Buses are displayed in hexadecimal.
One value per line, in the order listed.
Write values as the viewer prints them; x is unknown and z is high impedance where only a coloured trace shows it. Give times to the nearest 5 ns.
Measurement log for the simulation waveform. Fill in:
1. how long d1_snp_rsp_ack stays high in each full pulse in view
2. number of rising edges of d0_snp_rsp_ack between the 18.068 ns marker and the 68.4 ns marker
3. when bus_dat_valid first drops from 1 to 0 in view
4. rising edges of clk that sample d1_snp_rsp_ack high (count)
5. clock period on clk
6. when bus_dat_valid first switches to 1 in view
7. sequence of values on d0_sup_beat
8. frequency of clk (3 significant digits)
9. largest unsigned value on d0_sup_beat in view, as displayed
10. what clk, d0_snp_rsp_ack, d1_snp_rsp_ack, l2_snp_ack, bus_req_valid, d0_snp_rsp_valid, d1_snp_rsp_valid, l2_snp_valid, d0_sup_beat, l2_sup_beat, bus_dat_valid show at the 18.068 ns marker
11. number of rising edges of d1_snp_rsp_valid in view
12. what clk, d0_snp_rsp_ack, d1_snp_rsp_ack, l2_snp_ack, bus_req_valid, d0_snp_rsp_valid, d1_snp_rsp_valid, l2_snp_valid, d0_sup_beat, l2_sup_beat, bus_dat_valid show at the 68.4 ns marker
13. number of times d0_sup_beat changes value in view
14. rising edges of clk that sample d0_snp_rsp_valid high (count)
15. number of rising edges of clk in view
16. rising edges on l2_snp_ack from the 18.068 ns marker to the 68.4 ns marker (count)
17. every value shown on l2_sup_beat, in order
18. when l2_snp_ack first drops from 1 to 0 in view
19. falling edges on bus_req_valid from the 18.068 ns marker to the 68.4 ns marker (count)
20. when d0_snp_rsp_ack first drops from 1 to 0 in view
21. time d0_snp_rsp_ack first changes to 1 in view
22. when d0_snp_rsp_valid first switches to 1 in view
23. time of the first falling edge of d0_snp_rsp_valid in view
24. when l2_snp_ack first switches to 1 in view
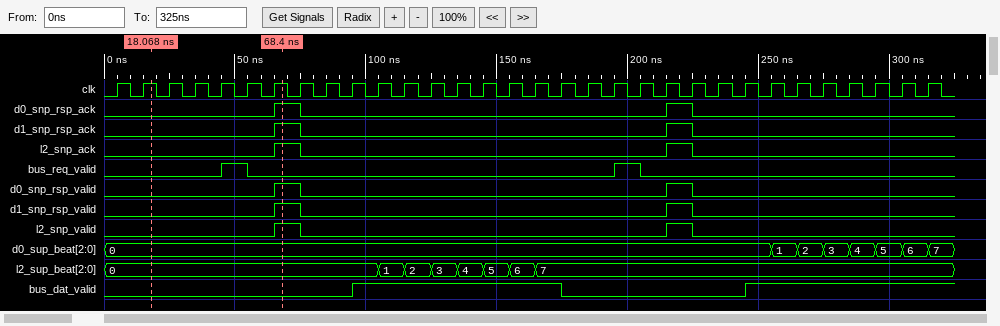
10 ns, 10 ns
1
175 ns
2
10 ns
95 ns
0, 1, 2, 3, 4, 5, 6, 7
100 MHz
7
clk=1, d0_snp_rsp_ack=0, d1_snp_rsp_ack=0, l2_snp_ack=0, bus_req_valid=0, d0_snp_rsp_valid=0, d1_snp_rsp_valid=0, l2_snp_valid=0, d0_sup_beat=0, l2_sup_beat=0, bus_dat_valid=0
2
clk=1, d0_snp_rsp_ack=1, d1_snp_rsp_ack=1, l2_snp_ack=1, bus_req_valid=0, d0_snp_rsp_valid=1, d1_snp_rsp_valid=1, l2_snp_valid=1, d0_sup_beat=0, l2_sup_beat=0, bus_dat_valid=0
7
2
32
1
0, 1, 2, 3, 4, 5, 6, 7
75 ns
1
75 ns
65 ns
65 ns
75 ns
65 ns
